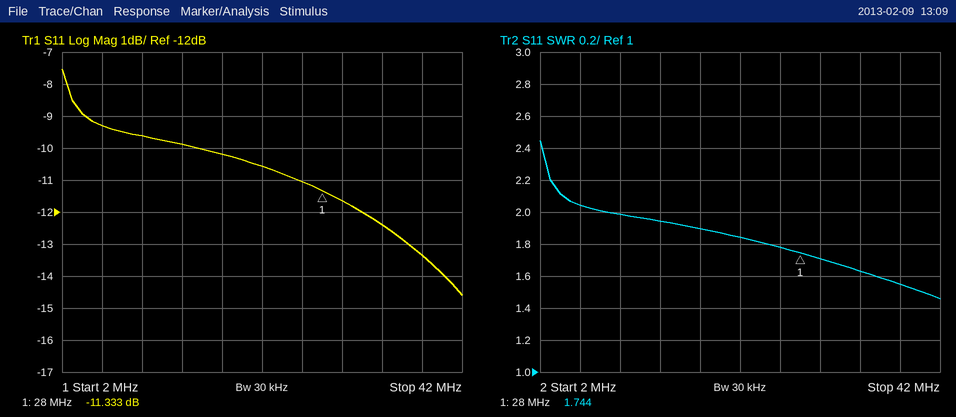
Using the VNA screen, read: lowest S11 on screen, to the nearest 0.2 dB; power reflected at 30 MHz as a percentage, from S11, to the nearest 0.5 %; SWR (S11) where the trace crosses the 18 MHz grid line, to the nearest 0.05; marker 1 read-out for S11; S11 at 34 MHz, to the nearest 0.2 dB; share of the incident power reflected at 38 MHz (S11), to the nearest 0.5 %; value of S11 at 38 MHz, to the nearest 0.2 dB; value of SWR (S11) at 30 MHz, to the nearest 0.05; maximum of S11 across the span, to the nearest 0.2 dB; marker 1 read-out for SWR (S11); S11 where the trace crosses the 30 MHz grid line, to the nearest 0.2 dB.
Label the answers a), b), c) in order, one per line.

a) -14.6 dB
b) 7.0 %
c) 1.90
d) -11.333 dB
e) -12.4 dB
f) 4.5 %
g) -13.4 dB
h) 1.70
i) -7.6 dB
j) 1.744
k) -11.6 dB
